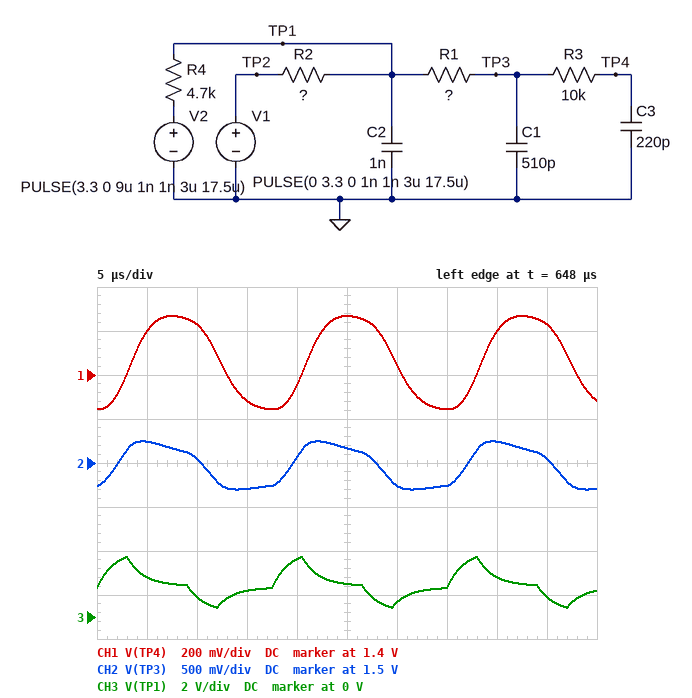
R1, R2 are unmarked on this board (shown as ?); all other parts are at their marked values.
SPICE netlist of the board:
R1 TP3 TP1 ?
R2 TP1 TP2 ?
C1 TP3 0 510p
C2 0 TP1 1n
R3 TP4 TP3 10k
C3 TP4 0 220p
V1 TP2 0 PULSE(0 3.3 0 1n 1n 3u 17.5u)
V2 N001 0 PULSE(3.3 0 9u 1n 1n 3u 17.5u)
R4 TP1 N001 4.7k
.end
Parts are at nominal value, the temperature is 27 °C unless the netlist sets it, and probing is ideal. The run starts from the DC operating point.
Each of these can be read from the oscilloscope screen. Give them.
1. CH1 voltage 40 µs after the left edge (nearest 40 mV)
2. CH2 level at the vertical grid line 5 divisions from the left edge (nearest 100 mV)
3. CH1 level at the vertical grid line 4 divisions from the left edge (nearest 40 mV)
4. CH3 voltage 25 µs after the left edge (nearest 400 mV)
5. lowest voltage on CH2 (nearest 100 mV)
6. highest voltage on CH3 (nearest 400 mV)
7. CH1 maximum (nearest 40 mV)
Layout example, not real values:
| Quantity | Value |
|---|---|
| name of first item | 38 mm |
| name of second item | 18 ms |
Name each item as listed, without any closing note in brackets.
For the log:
| Quantity | Value |
|---|---|
| CH1 voltage 40 µs after the left edge | 1.60 V |
| CH2 level at the vertical grid line 5 divisions from the left edge | 1.7 V |
| CH1 level at the vertical grid line 4 divisions from the left edge | 1.36 V |
| CH3 voltage 25 µs after the left edge | 1.6 V |
| lowest voltage on CH2 | 1.2 V |
| highest voltage on CH3 | 2.8 V |
| CH1 maximum | 1.68 V |
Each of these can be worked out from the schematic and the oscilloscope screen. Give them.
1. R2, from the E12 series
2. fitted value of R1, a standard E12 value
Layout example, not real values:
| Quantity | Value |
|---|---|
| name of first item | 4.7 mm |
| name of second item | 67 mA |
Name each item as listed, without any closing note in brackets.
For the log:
| Quantity | Value |
|---|---|
| R2, from the E12 series | 3.3 kΩ |
| fitted value of R1, a standard E12 value | 10 kΩ |
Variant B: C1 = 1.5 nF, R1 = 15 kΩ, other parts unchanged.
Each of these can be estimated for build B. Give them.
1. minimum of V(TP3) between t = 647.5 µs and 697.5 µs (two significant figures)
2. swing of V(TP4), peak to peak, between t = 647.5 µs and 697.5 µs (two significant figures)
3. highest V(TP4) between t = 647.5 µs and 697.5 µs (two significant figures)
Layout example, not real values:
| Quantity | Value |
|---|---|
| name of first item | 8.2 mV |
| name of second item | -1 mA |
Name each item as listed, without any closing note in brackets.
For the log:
| Quantity | Value |
|---|---|
| minimum of V(TP3) between t = 647.5 µs and 697.5 µs | 1.4 V |
| swing of V(TP4), peak to peak, between t = 647.5 µs and 697.5 µs | 140 mV |
| highest V(TP4) between t = 647.5 µs and 697.5 µs | 1.5 V |
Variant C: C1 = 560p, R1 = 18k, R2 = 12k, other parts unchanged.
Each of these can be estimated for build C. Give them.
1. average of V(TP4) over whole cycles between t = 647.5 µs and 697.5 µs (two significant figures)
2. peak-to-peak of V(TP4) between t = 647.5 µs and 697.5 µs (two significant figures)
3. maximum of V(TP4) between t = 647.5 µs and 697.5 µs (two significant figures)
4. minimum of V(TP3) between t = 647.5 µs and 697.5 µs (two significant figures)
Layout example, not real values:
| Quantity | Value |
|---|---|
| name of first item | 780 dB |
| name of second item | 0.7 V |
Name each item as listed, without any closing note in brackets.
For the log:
| Quantity | Value |
|---|---|
| average of V(TP4) over whole cycles between t = 647.5 µs and 697.5 µs | 2.1 V |
| peak-to-peak of V(TP4) between t = 647.5 µs and 697.5 µs | 210 mV |
| maximum of V(TP4) between t = 647.5 µs and 697.5 µs | 2.2 V |
| minimum of V(TP3) between t = 647.5 µs and 697.5 µs | 2.0 V |
